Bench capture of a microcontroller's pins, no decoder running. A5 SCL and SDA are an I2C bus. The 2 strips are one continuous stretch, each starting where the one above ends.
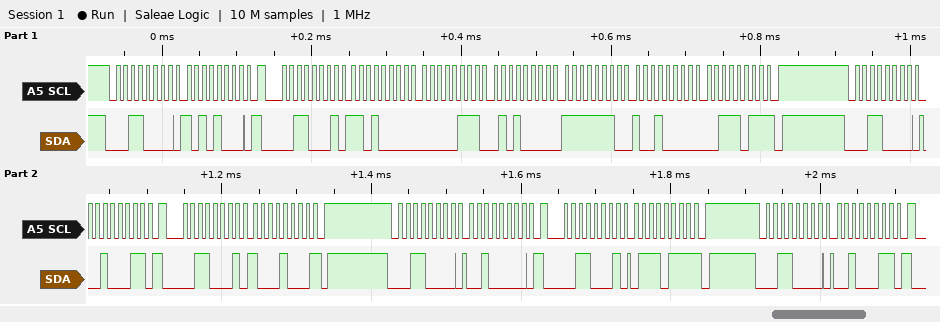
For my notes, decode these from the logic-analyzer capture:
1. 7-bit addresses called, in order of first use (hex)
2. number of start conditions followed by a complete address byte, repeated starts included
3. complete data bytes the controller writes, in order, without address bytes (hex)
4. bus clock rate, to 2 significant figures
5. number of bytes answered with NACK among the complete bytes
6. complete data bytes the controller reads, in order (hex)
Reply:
0x18
7
A8 23 20 23
100 kHz
3
D0 07 50 FE 90 3B 88 77
